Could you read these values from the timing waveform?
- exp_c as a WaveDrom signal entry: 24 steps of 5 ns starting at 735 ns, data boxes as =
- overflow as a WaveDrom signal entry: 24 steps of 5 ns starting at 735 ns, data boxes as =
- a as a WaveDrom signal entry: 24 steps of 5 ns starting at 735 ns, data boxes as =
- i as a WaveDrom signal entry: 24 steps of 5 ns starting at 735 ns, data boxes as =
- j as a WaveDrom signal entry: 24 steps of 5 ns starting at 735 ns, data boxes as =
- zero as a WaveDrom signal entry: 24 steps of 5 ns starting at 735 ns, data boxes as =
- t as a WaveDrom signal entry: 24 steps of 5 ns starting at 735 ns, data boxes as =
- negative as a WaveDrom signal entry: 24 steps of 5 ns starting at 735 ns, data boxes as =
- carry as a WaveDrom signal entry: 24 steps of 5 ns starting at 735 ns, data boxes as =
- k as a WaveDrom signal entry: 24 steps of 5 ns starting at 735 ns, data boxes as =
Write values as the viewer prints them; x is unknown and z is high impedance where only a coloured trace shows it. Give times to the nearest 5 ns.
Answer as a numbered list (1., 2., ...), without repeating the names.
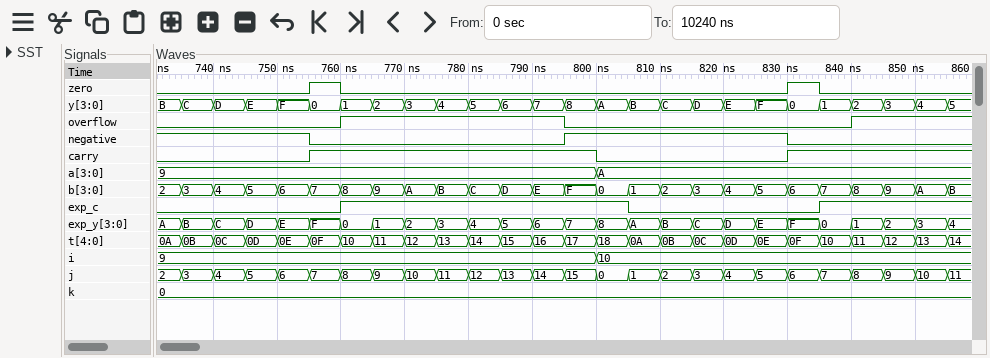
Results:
1. {name: 'exp_c', wave: '0....1........0.....1...'}
2. {name: 'overflow', wave: '0....1......0........1..'}
3. {name: 'a', wave: '=............=..........', data: '9 A'}
4. {name: 'i', wave: '=............=..........', data: '9 10'}
5. {name: 'j', wave: '========================', data: '3 4 5 6 7 8 9 10 11 12 13 14 15 0 1 2 3 4 5 6 7 8 9 10'}
6. {name: 'zero', wave: '0...10.............10...'}
7. {name: 't', wave: '========================', data: '0B 0C 0D 0E 0F 10 11 12 13 14 15 16 17 18 0A 0B 0C 0D 0E 0F 10 11 12 13'}
8. {name: 'negative', wave: '1...0.......1......0....'}
9. {name: 'carry', wave: '0...1........0.....1....'}
10. {name: 'k', wave: '=.......................', data: '0'}
